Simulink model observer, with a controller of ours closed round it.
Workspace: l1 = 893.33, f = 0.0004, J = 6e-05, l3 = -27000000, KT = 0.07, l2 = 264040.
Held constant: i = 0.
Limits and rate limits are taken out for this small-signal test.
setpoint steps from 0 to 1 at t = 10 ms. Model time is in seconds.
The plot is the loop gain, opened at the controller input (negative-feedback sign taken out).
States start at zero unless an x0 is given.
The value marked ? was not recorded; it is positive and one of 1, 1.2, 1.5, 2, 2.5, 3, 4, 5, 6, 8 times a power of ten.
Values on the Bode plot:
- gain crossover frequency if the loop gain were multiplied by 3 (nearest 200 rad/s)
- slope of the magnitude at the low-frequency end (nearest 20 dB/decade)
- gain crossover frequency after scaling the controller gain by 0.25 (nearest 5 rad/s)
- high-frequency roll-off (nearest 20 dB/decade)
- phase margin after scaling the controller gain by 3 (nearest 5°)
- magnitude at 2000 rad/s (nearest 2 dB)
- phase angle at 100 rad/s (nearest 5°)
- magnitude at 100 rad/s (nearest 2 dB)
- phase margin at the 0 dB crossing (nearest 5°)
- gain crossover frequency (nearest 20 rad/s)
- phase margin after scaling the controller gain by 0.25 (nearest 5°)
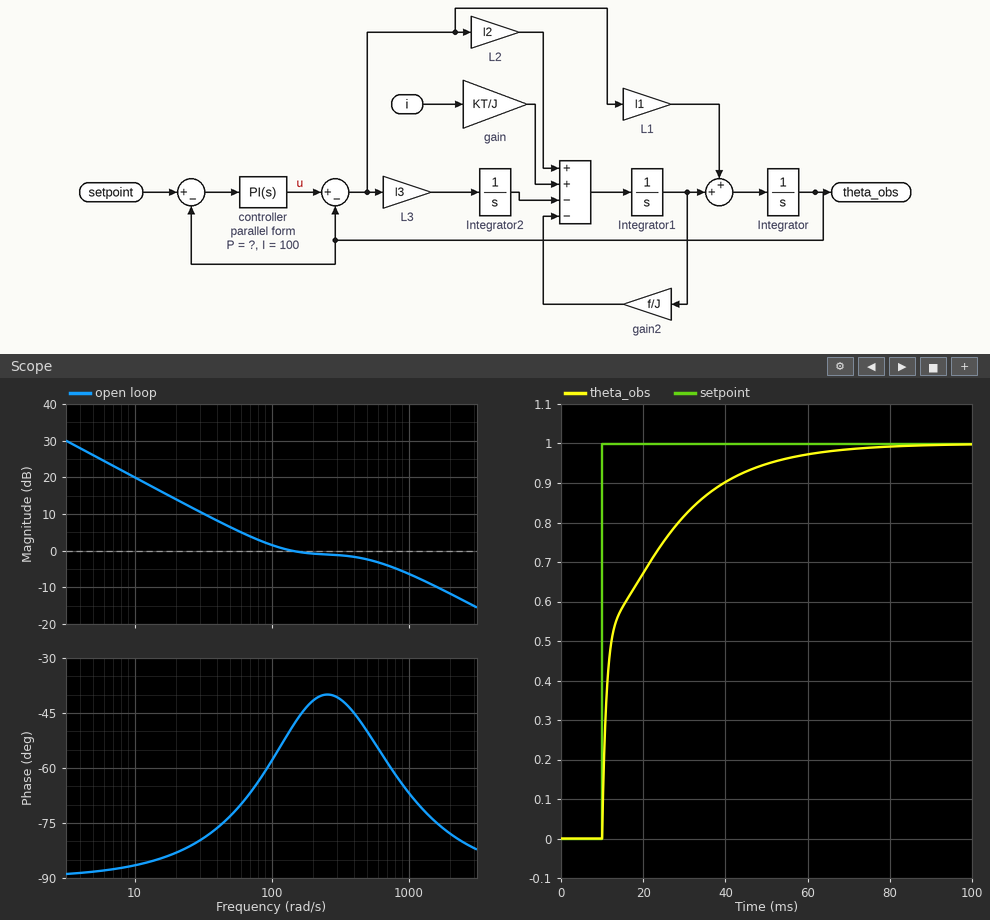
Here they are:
1600 rad/s
-20 dB/decade
25 rad/s
-20 dB/decade
105°
-12 dB
-60°
2 dB
130°
140 rad/s
100°
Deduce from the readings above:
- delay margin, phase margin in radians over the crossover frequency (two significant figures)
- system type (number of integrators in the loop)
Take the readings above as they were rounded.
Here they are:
0.016 s
1
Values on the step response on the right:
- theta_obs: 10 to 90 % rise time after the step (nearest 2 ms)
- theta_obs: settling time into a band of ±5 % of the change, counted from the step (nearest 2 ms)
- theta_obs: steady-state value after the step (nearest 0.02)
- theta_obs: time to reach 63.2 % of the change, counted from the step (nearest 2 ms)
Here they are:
30 ms
40 ms
1.00
8 ms
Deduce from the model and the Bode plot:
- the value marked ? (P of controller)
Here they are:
0.6
